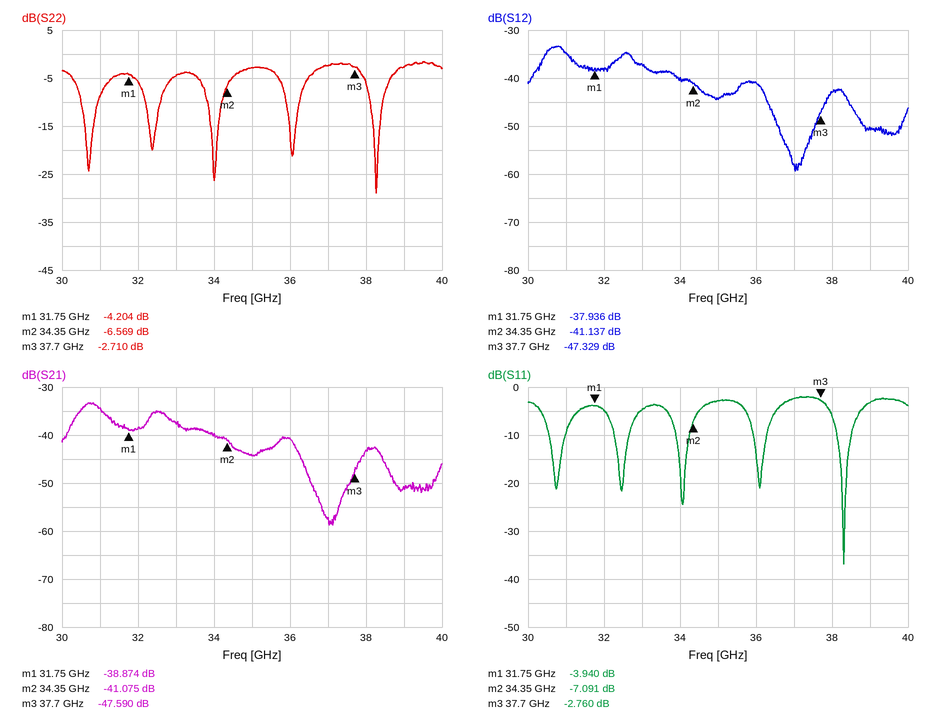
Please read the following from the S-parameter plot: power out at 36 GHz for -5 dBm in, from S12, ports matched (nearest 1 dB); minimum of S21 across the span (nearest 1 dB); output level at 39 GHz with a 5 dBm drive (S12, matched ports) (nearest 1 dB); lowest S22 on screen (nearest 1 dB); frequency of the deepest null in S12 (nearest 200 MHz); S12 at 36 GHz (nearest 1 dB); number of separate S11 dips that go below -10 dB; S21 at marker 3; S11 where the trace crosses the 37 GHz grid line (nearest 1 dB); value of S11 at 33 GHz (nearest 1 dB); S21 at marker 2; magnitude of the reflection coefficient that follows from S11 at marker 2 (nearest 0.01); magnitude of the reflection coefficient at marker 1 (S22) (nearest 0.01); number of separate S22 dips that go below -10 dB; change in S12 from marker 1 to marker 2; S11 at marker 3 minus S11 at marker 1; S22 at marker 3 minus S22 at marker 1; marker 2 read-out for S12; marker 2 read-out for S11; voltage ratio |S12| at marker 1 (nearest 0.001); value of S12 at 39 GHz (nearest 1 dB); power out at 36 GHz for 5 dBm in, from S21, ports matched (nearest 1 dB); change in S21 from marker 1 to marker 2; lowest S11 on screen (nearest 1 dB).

-46 dBm
-59 dB
-45 dBm
-29 dB
37.0 GHz
-41 dB
5
-47.590 dB
-2 dB
-5 dB
-41.075 dB
0.44
0.62
5
-3.201 dB
1.180 dB
1.494 dB
-41.137 dB
-7.091 dB
0.013
-50 dB
-36 dBm
-2.201 dB
-37 dB
